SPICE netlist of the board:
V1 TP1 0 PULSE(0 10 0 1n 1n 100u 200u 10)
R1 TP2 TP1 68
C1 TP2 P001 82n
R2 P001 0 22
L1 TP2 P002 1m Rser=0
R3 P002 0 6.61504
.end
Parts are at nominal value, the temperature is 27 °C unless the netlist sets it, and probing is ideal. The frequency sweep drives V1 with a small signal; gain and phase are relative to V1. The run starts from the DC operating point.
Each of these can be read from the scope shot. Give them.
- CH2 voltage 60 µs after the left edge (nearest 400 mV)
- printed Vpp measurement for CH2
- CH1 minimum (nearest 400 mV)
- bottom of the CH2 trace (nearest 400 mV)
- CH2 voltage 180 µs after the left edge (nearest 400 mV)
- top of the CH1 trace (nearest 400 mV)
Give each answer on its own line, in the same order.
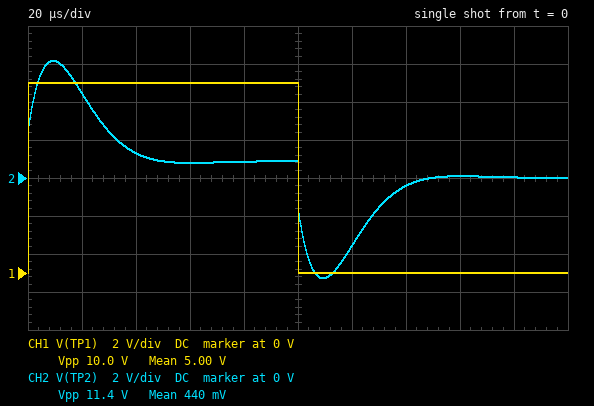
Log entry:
800 mV
11.4 V
0 V
-5.2 V
0 V
10.0 V
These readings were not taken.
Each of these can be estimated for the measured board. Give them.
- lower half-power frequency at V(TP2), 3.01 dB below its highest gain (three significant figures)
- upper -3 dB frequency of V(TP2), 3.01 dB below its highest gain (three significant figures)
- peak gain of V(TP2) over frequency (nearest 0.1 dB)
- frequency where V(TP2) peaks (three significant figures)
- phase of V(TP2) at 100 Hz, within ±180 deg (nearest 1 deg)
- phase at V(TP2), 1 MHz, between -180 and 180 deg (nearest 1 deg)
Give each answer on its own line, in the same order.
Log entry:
7.81 kHz
35.4 kHz
-1.2 dB
16.3 kHz
5 deg
-4 deg
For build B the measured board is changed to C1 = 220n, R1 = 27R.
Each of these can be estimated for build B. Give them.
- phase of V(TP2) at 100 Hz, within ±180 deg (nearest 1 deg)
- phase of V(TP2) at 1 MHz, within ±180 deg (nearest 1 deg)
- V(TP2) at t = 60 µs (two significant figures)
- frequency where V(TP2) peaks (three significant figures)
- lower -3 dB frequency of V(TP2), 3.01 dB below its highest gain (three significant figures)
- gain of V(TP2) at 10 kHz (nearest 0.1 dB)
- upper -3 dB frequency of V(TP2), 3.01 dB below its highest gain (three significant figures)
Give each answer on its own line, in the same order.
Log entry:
4 deg
-1 deg
3.3 V
9.48 kHz
3.68 kHz
-1.2 dB
29.8 kHz
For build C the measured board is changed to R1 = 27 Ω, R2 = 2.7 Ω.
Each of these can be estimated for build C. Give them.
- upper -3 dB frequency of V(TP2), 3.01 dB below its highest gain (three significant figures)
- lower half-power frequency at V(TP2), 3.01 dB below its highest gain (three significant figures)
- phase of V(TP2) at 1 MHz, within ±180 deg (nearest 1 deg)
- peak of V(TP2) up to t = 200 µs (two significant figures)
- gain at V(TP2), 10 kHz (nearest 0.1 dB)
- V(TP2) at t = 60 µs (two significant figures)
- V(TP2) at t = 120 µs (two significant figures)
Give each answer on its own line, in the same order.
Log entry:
72.1 kHz
4.69 kHz
-32 deg
8.7 V
-0.7 dB
3.1 V
-4.5 V
